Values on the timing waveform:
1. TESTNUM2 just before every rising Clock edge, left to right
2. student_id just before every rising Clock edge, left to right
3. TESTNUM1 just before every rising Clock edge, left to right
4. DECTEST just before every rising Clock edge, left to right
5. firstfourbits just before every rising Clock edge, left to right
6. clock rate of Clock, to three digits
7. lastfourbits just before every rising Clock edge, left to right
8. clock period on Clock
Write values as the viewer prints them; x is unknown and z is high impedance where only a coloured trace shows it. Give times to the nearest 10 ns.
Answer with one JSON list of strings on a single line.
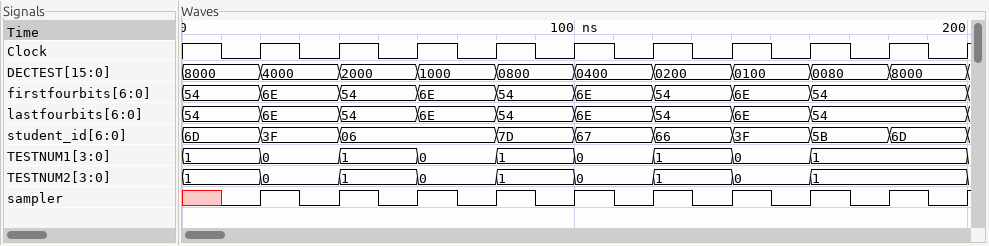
["1, 0, 1, 0, 1, 0, 1, 0, 1, 1", "6D, 3F, 06, 06, 7D, 67, 66, 3F, 5B, 6D", "1, 0, 1, 0, 1, 0, 1, 0, 1, 1", "8000, 4000, 2000, 1000, 0800, 0400, 0200, 0100, 0080, 8000", "54, 6E, 54, 6E, 54, 6E, 54, 6E, 54, 54", "50.0 MHz", "54, 6E, 54, 6E, 54, 6E, 54, 6E, 54, 54", "20 ns"]
